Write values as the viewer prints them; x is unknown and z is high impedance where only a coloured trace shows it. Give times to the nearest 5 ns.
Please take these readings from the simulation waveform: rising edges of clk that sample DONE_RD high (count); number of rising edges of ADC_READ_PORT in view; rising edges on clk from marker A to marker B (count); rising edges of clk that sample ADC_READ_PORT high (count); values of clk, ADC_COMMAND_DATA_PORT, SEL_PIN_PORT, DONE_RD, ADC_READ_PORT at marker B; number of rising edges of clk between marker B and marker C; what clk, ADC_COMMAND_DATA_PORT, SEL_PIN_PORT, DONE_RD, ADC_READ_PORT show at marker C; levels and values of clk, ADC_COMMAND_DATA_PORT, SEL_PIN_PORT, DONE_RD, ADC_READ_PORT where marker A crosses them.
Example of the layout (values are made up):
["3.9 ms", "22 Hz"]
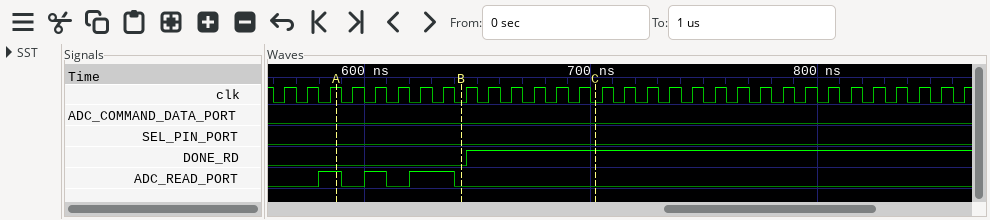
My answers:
["22", "3", "5", "4", "clk=0, ADC_COMMAND_DATA_PORT=0, SEL_PIN_PORT=0, DONE_RD=0, ADC_READ_PORT=0", "6", "clk=0, ADC_COMMAND_DATA_PORT=0, SEL_PIN_PORT=0, DONE_RD=1, ADC_READ_PORT=0", "clk=1, ADC_COMMAND_DATA_PORT=0, SEL_PIN_PORT=0, DONE_RD=0, ADC_READ_PORT=1"]
